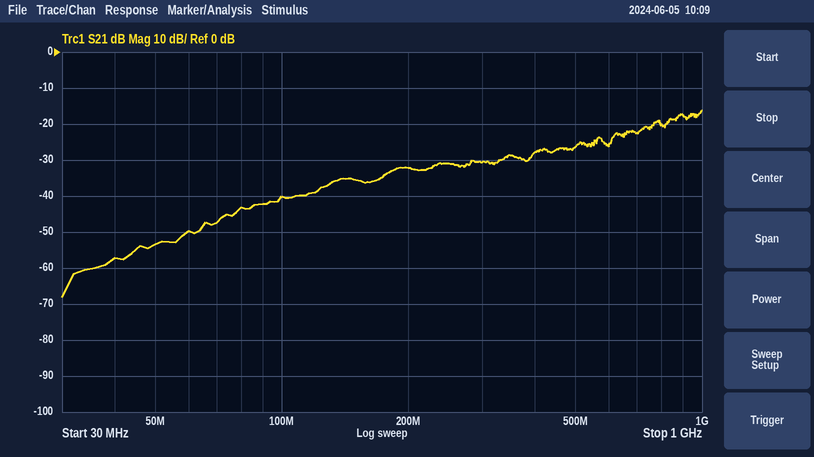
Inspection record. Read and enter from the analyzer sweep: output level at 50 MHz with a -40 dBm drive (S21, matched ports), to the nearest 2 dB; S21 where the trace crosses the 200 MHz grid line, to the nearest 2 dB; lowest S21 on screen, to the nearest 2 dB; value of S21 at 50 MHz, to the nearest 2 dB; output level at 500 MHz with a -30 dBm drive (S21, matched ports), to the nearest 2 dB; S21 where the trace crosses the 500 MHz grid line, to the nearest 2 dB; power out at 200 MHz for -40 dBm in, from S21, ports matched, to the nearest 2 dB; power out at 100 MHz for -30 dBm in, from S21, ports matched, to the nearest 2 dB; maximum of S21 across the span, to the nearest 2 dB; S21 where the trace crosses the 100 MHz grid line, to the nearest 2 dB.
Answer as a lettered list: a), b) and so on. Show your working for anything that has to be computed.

a) -40 dBm + (-54 dB) = -94 dBm
b) -32 dB
c) -68 dB
d) -54 dB
e) -30 dBm + (-26 dB) = -56 dBm
f) -26 dB
g) -40 dBm + (-32 dB) = -72 dBm
h) -30 dBm + (-40 dB) = -70 dBm
i) -16 dB
j) -40 dB
